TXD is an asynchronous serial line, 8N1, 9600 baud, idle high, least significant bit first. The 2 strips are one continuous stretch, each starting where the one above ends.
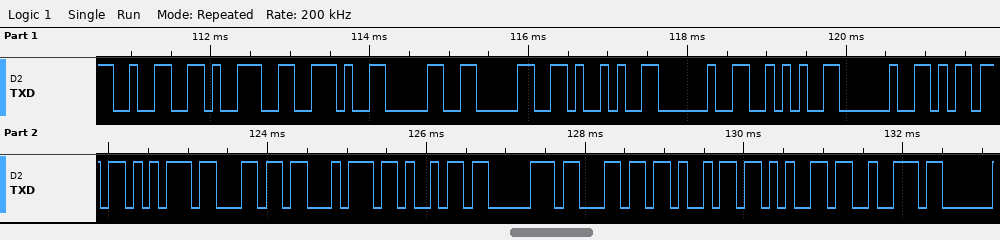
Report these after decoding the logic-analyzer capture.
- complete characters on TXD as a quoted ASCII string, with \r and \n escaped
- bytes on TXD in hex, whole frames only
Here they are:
"29.00) * multiplier"
32 39 2E 30 30 29 20 2A 20 6D 75 6C 74 69 70 6C 69 65 72
